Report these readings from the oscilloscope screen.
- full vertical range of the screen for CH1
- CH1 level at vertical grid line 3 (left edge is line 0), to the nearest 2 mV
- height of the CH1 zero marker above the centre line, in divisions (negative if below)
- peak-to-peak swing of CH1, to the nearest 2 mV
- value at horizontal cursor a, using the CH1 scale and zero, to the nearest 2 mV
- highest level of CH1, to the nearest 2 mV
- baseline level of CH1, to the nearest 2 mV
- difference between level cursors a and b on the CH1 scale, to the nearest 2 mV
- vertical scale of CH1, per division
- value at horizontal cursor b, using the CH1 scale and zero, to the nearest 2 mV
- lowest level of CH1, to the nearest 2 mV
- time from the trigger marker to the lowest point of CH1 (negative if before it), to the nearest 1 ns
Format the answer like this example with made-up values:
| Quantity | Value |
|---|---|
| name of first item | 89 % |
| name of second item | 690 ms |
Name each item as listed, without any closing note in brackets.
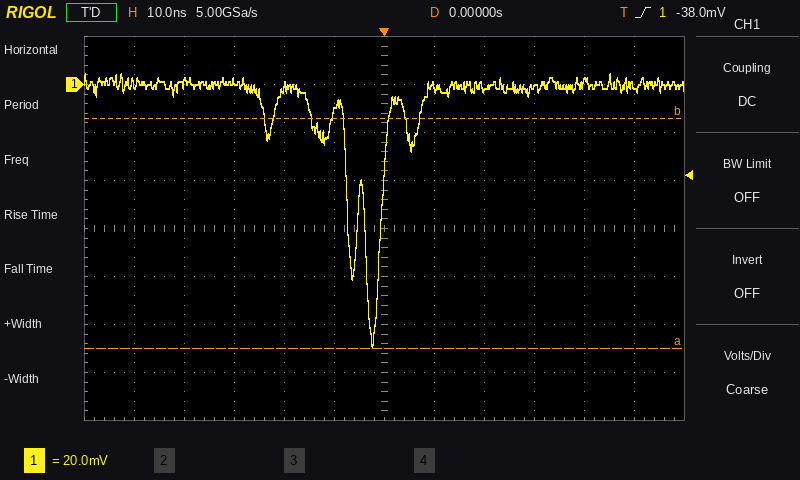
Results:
| Quantity | Value |
|---|---|
| full vertical range of the screen for CH1 | 160 mV |
| CH1 level at vertical grid line 3 (left edge is line 0), to the nearest 2 mV | 2 mV |
| height of the CH1 zero marker above the centre line, in divisions | +3.0 div |
| peak-to-peak swing of CH1, to the nearest 2 mV | 114 mV |
| value at horizontal cursor a, using the CH1 scale and zero, to the nearest 2 mV | -110 mV |
| highest level of CH1, to the nearest 2 mV | 4 mV |
| baseline level of CH1, to the nearest 2 mV | 0 mV |
| difference between level cursors a and b on the CH1 scale, to the nearest 2 mV | 96 mV |
| vertical scale of CH1, per division | 20 mV |
| value at horizontal cursor b, using the CH1 scale and zero, to the nearest 2 mV | -14 mV |
| lowest level of CH1, to the nearest 2 mV | -110 mV |
| time from the trigger marker to the lowest point of CH1 (negative if before it), to the nearest 1 ns | -2 ns |
